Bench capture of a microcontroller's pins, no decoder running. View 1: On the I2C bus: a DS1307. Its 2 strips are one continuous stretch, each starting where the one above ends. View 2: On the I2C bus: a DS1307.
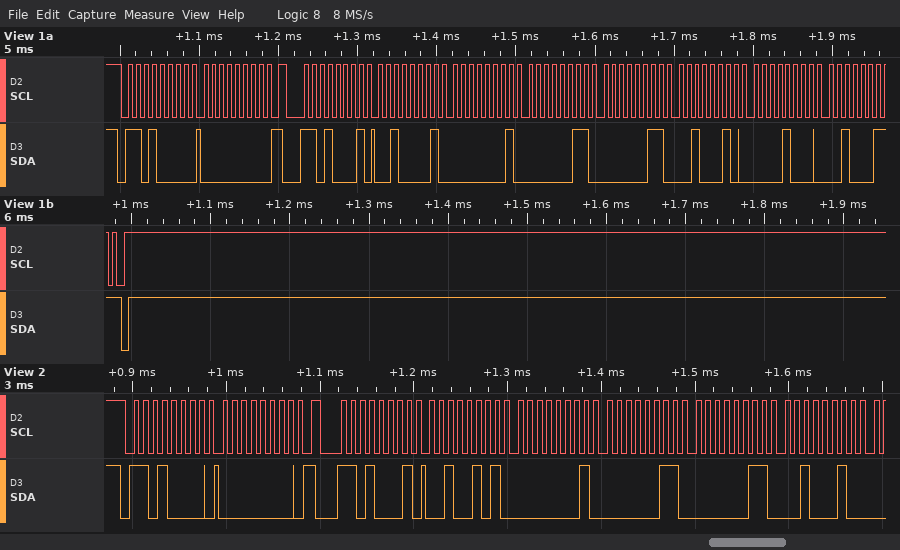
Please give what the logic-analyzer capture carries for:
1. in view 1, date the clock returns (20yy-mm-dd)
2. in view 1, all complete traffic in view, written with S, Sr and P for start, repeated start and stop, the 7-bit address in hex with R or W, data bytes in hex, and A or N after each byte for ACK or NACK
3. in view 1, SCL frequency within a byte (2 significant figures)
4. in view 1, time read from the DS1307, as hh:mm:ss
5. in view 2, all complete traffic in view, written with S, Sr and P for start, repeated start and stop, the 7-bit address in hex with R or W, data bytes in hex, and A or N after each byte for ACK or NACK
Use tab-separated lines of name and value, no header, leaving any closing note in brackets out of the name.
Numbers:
in view 1, date the clock returns	2023-08-22
in view 1, all complete traffic in view, written with S, Sr and P for start, repeated start and stop, the 7-bit address in hex with R or W, data bytes in hex, and A or N after each byte for ACK or NACK	S 68W A 00 A Sr 68R A 21 A 01 A 03 A 03 A 22 A 08 A 23 N P
in view 1, SCL frequency within a byte	100 kHz
in view 1, time read from the DS1307, as hh:mm:ss	03:01:21
in view 2, all complete traffic in view, written with S, Sr and P for start, repeated start and stop, the 7-bit address in hex with R or W, data bytes in hex, and A or N after each byte for ACK or NACK	S 68W A 00 A Sr 68R A 25 A 01 A 03 A 03 A 22 A
